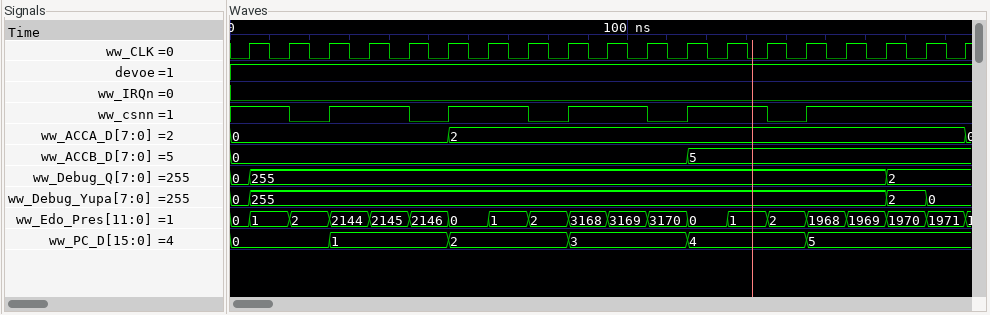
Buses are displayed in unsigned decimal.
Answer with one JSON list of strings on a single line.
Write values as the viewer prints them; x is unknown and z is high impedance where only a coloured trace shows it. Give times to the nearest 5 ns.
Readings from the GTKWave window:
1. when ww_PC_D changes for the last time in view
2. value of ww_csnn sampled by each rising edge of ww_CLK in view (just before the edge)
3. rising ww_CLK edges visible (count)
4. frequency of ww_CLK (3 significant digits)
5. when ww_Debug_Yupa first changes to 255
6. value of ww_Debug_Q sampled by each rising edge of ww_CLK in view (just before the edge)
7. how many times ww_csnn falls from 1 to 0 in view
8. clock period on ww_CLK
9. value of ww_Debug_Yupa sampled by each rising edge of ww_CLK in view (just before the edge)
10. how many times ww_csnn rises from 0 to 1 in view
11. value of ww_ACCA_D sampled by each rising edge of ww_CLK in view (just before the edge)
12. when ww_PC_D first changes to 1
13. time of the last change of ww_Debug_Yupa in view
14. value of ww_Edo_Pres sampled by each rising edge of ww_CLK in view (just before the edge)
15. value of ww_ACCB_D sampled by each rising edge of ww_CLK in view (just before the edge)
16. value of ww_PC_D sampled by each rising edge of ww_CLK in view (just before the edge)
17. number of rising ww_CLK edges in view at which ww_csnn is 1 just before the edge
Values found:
["145 ns", "1 1 0 1 1 0 1 1 0 1 1 0 1 1 0 1 1 1 1", "19", "100 MHz", "5 ns", "0, 255, 255, 255, 255, 255, 255, 255, 255, 255, 255, 255, 255, 255, 255, 255, 255, 2, 2", "5", "10 ns", "0, 255, 255, 255, 255, 255, 255, 255, 255, 255, 255, 255, 255, 255, 255, 255, 255, 2, 0", "5", "0, 0, 0, 0, 0, 0, 2, 2, 2, 2, 2, 2, 2, 2, 2, 2, 2, 2, 2", "25 ns", "175 ns", "0, 1, 2, 2144, 2145, 2146, 0, 1, 2, 3168, 3169, 3170, 0, 1, 2, 1968, 1969, 1970, 1971", "0, 0, 0, 0, 0, 0, 0, 0, 0, 0, 0, 0, 5, 5, 5, 5, 5, 5, 5", "0, 0, 0, 1, 1, 1, 2, 2, 2, 3, 3, 3, 4, 4, 4, 5, 5, 5, 5", "14"]
